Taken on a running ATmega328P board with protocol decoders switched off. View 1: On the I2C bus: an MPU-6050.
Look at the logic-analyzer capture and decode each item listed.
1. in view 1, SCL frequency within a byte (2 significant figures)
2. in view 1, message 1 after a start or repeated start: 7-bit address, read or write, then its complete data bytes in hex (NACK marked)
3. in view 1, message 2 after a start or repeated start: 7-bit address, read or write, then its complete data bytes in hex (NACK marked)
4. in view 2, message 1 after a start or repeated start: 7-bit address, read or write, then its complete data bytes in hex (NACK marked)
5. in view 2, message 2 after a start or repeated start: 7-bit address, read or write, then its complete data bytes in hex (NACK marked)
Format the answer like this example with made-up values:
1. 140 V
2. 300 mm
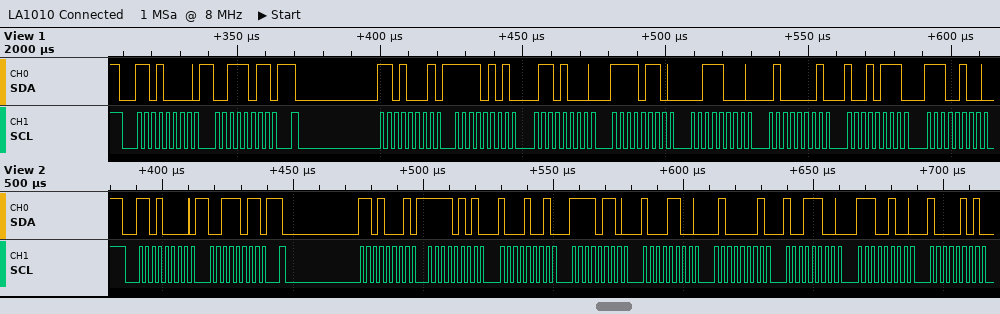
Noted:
1. 400 kHz
2. 0x68 write: 3B
3. 0x68 read: F5 68 F6 38 41 97 E4
4. 0x68 write: 3B
5. 0x68 read: F5 89 F6 8C 41 9C E4 85
